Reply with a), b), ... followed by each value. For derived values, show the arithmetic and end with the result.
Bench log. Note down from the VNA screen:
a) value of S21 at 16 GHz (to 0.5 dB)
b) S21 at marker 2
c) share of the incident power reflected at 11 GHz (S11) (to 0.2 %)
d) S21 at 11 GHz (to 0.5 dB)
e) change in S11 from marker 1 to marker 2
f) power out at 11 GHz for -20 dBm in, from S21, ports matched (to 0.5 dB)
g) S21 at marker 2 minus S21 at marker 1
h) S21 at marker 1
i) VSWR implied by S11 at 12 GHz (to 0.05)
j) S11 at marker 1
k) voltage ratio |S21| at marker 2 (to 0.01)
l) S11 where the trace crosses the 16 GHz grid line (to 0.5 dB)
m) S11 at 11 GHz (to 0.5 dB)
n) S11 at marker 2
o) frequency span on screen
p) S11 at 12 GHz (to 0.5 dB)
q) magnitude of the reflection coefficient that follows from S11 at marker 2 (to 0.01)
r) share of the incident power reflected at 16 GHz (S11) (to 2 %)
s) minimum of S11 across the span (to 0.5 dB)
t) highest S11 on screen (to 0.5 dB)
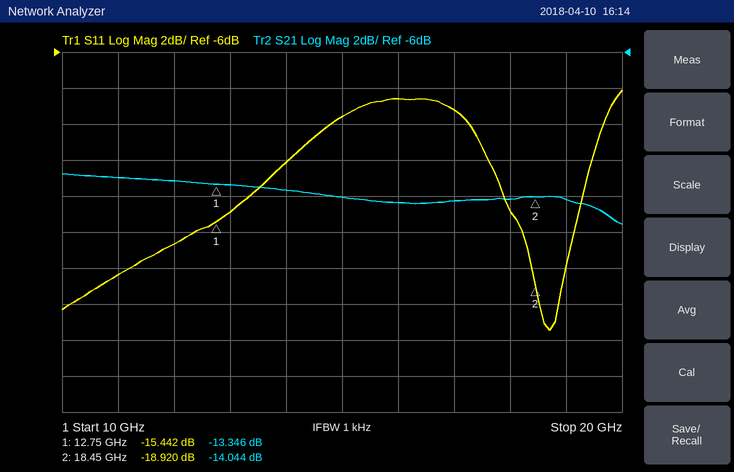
a) -14.5 dB
b) -14.044 dB
c) 10^(-18.5/10) ≈ 1.4 %
d) -13.0 dB
e) -18.92 − (-15.442) = -3.478 dB
f) -20 dBm + (-13.0 dB) = -33.0 dBm
g) -14.044 − (-13.346) = -0.698 dB
h) -13.346 dB
i) |Γ| = 10^(-16.5/20) = 0.1496; VSWR = (1 + 0.1496)/(1 − 0.1496) ≈ 1.35
j) -15.442 dB
k) 10^(-14.044/20) ≈ 0.20
l) -8.5 dB
m) -18.5 dB
n) -18.920 dB
o) 10 GHz
p) -16.5 dB
q) 10^(-18.92/20) ≈ 0.11
r) 10^(-8.5/10) ≈ 14 %
s) -21.5 dB
t) -8.0 dB
